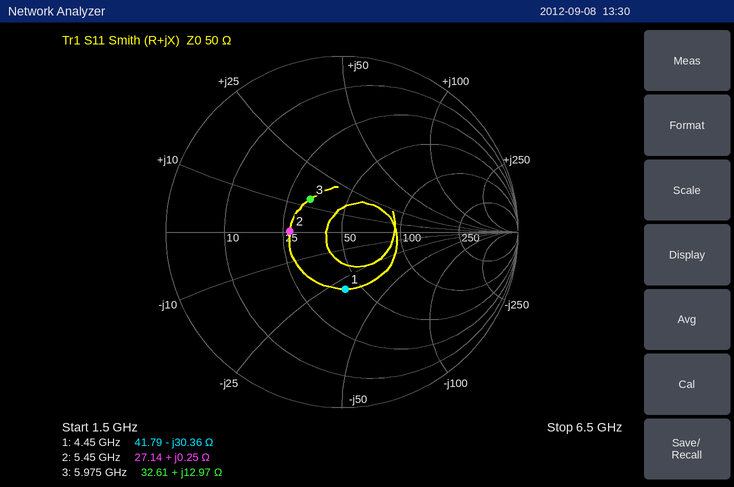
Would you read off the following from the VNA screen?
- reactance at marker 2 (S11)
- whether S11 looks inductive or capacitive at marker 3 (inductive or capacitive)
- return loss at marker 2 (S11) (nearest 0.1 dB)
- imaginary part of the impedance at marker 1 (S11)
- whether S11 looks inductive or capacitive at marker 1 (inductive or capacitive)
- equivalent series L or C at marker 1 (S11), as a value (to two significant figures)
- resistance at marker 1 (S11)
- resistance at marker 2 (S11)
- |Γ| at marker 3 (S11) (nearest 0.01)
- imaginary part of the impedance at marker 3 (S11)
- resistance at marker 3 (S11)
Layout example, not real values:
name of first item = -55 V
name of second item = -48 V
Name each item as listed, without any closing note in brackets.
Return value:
reactance at marker 2 = +0.25 Ω
whether S11 looks inductive or capacitive at marker 3 = inductive
return loss at marker 2 (S11) = 10.6 dB
imaginary part of the impedance at marker 1 = -30.36 Ω
whether S11 looks inductive or capacitive at marker 1 = capacitive
equivalent series L or C at marker 1 (S11), as a value = 1.2 pF
resistance at marker 1 = 41.79 Ω
resistance at marker 2 = 27.14 Ω
|Γ| at marker 3 (S11) = 0.26
imaginary part of the impedance at marker 3 = +12.97 Ω
resistance at marker 3 = 32.61 Ω
